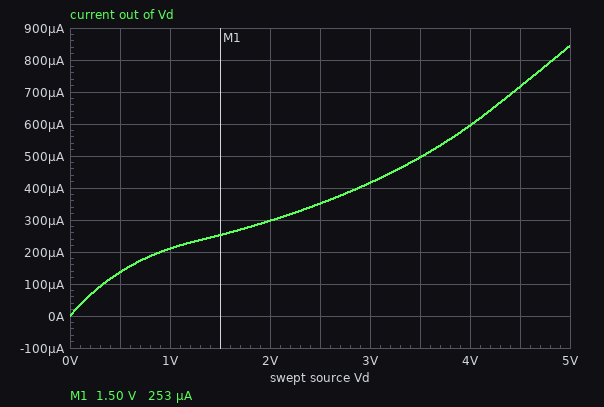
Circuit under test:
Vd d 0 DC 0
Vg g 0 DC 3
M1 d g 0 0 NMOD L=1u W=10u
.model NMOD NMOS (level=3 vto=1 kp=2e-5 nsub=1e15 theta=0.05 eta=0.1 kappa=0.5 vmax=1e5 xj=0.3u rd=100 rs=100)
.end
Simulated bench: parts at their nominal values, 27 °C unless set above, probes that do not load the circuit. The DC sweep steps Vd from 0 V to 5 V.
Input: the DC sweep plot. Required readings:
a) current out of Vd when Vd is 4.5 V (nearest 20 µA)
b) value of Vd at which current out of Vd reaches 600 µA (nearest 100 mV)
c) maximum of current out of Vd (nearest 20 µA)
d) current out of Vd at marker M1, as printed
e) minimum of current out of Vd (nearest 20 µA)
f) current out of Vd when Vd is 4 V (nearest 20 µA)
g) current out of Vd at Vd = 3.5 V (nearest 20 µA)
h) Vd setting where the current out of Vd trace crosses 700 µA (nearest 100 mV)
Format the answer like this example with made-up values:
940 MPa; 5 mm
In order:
720 µA; 4.0 V; 840 µA; 253 µA; 0 A; 600 µA; 500 µA; 4.4 V
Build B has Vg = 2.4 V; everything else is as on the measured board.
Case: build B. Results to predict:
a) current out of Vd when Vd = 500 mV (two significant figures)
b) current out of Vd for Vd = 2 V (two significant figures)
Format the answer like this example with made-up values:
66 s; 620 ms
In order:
100 µA; 210 µA
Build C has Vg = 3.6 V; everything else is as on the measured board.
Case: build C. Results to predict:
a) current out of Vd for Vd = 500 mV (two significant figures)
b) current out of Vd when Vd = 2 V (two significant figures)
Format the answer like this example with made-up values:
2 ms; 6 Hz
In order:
170 µA; 380 µA
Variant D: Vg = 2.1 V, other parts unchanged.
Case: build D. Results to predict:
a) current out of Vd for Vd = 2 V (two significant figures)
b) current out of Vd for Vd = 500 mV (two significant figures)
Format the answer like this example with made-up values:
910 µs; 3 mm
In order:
170 µA; 80 µA
